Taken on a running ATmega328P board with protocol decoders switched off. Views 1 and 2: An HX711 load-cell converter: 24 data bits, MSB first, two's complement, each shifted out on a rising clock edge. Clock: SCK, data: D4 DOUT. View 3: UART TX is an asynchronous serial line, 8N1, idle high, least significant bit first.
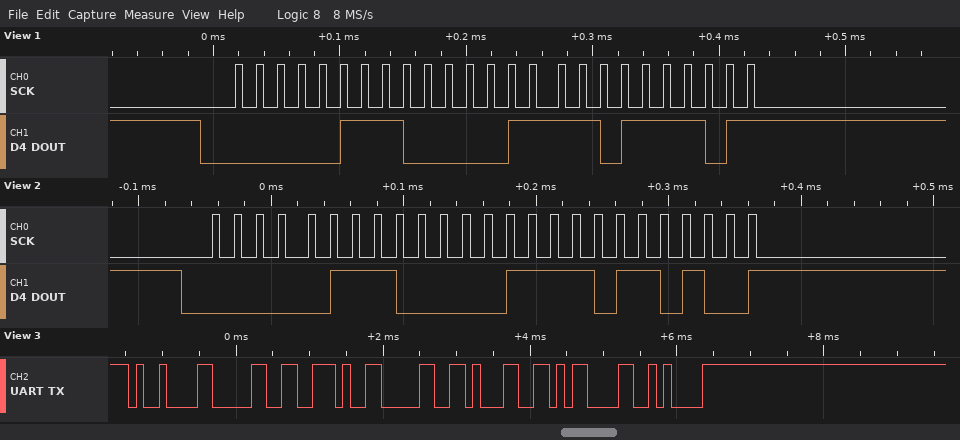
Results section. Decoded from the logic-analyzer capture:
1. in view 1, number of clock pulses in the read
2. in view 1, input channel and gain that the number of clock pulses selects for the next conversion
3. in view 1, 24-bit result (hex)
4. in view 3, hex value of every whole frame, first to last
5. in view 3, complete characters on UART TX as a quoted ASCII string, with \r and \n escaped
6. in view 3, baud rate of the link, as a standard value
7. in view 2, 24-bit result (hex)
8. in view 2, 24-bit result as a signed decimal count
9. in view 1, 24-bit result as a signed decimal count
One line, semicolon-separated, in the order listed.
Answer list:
25; channel A, gain 128; 0x0707BD; 09 30 2E 30 31 0D 0A; "\t0.01\r\n"; 9600 baud; 0x0707B4; 460724; 460733
